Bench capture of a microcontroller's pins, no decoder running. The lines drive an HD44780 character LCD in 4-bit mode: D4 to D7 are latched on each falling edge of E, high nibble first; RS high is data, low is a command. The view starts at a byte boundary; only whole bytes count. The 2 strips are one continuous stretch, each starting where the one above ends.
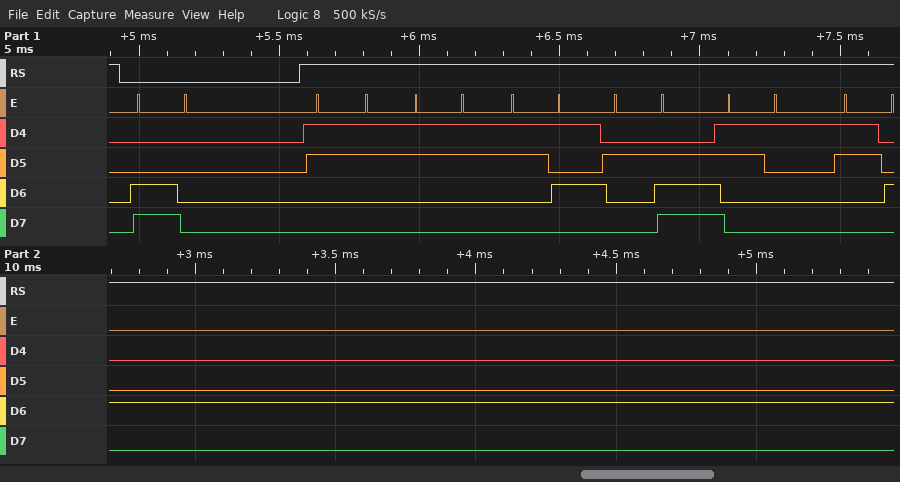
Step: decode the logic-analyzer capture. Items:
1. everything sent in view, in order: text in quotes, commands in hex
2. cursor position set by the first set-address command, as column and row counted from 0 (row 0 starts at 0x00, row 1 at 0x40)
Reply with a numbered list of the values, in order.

1. 0xC0 "335.14"
2. column 0, row 1
